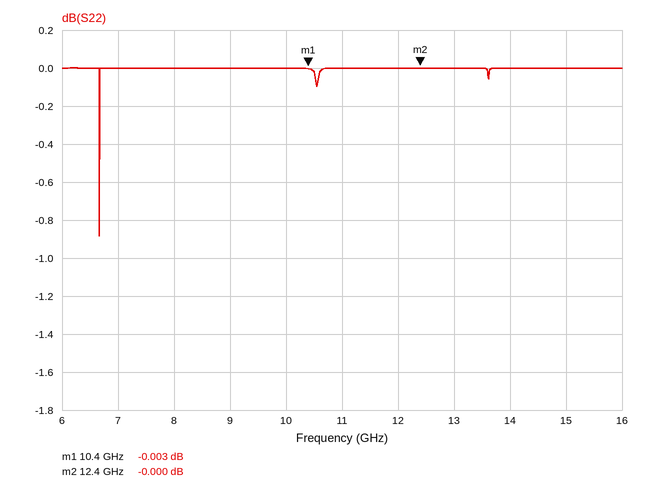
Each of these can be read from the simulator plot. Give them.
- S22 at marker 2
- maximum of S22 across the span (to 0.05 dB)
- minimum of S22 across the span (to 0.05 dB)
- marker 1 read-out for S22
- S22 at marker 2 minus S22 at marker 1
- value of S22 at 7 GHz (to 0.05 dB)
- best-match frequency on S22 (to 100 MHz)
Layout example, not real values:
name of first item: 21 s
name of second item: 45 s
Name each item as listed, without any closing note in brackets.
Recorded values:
S22 at marker 2: -0.000 dB
maximum of S22 across the span: 0.00 dB
minimum of S22 across the span: -0.90 dB
marker 1 read-out for S22: -0.003 dB
S22 at marker 2 minus S22 at marker 1: 0.003 dB
value of S22 at 7 GHz: 0.00 dB
best-match frequency on S22: 6.7 GHz
